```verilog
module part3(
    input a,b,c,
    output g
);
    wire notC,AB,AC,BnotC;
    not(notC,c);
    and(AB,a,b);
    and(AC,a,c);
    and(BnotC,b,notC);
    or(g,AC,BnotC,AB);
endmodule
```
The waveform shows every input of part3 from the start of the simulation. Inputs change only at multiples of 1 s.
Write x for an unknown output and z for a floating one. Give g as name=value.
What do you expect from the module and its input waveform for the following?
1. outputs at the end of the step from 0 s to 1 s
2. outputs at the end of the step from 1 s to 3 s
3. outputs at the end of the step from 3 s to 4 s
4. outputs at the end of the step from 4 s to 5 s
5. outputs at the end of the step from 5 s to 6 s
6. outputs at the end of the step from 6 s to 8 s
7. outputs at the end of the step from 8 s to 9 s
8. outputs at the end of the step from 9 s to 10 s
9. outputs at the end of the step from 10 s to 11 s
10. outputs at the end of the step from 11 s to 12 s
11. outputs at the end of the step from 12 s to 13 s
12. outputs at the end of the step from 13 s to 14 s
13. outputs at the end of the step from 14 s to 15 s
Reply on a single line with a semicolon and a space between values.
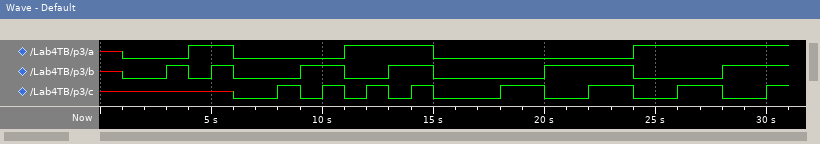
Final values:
g=x; g=0; g=x; g=x; g=1; g=0; g=0; g=1; g=0; g=0; g=1; g=1; g=1
